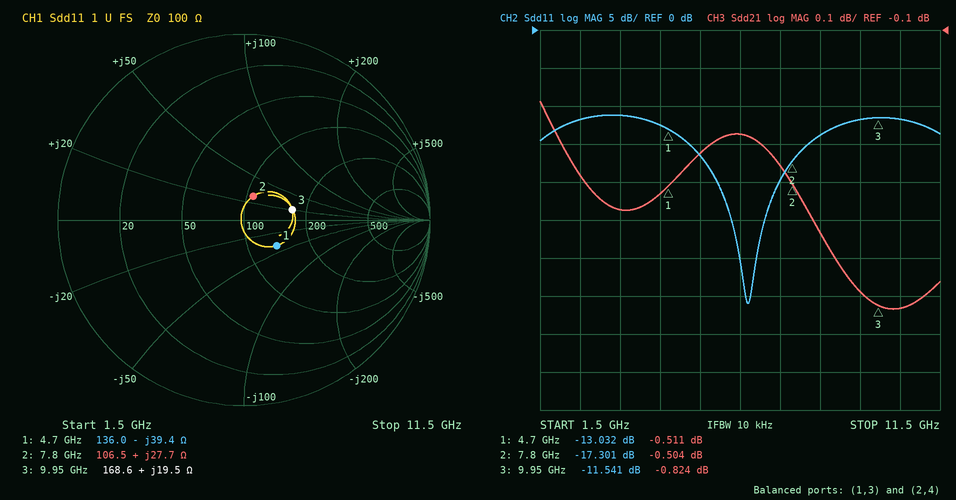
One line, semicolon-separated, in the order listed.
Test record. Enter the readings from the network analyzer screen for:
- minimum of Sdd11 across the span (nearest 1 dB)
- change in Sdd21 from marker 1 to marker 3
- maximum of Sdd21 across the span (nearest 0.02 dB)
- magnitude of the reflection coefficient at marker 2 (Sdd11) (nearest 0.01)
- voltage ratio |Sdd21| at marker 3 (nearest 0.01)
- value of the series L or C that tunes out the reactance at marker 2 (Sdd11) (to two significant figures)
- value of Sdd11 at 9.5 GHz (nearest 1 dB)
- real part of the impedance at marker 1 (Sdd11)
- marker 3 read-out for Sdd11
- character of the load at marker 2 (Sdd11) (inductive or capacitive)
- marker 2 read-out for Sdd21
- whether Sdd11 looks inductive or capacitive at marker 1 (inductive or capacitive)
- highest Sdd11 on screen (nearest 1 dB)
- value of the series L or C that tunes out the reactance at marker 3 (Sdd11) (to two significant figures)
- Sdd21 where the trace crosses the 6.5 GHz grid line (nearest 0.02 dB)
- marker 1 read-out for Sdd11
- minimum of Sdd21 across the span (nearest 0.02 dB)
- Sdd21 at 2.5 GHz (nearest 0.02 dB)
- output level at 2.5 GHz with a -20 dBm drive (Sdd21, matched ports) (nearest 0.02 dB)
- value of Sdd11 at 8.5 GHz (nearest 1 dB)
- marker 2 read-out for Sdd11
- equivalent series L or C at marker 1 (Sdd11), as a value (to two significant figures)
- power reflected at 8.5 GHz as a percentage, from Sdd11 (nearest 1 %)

-36 dB; -0.313 dB; -0.28 dB; 0.14; 0.91; 740 fF; -12 dB; 136.0 Ω; -11.541 dB; inductive; -0.504 dB; capacitive; -11 dB; 820 fF; -0.38 dB; -13.032 dB; -0.84 dB; -0.48 dB; -20.48 dBm; -14 dB; -17.301 dB; 860 fF; 4 %
